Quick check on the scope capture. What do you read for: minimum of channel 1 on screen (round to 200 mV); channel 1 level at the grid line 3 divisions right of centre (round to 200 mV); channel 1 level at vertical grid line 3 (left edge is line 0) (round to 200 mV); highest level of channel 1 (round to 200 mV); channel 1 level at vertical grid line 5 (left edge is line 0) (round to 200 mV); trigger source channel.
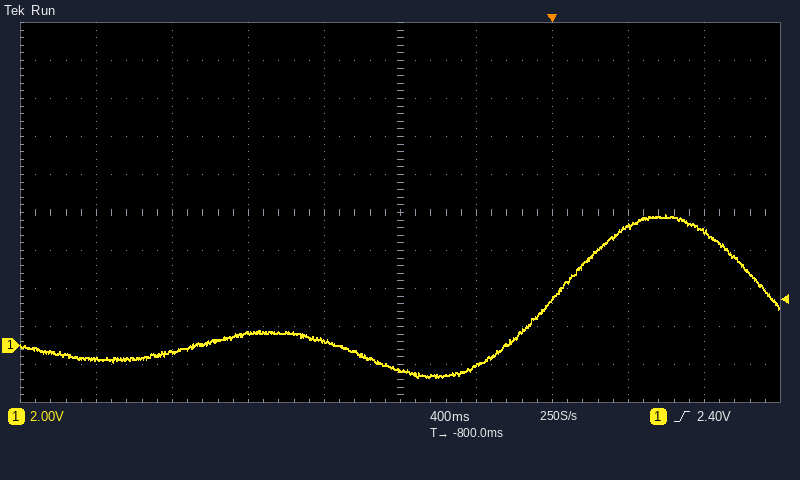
-1.6 V
6.2 V
600 mV
6.8 V
-1.2 V
channel 1
